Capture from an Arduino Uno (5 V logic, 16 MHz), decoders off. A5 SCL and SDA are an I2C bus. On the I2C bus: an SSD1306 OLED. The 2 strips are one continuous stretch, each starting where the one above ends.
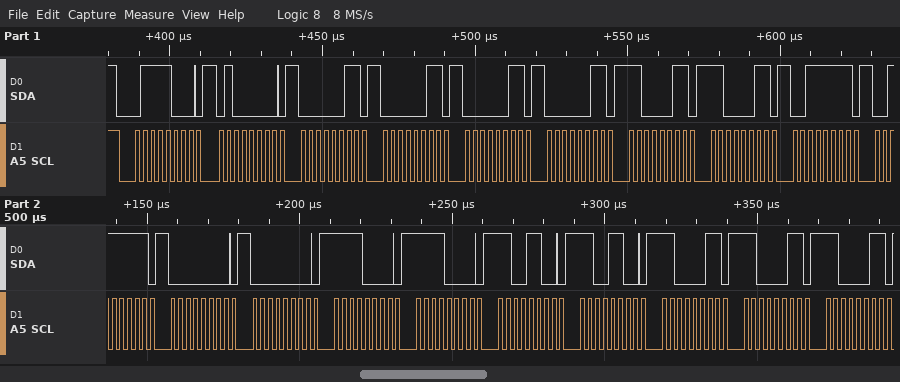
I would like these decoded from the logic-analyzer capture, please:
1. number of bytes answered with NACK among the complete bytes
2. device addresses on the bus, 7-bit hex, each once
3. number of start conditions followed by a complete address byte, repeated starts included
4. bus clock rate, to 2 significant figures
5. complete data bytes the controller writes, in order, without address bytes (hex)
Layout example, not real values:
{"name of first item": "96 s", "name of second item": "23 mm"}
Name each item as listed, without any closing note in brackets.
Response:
{"number of bytes answered with NACK among the complete bytes": "0", "device addresses on the bus, 7-bit hex, each once": "0x3C", "number of start conditions followed by a complete address byte, repeated starts included": "1", "bus clock rate, to 2 significant figures": "400 kHz", "complete data bytes the controller writes, in order, without address bytes": "40 03 03 03 03 C3 C3 3F 3F 00 00 F0 F0 CC CC C3 C3 C3"}
